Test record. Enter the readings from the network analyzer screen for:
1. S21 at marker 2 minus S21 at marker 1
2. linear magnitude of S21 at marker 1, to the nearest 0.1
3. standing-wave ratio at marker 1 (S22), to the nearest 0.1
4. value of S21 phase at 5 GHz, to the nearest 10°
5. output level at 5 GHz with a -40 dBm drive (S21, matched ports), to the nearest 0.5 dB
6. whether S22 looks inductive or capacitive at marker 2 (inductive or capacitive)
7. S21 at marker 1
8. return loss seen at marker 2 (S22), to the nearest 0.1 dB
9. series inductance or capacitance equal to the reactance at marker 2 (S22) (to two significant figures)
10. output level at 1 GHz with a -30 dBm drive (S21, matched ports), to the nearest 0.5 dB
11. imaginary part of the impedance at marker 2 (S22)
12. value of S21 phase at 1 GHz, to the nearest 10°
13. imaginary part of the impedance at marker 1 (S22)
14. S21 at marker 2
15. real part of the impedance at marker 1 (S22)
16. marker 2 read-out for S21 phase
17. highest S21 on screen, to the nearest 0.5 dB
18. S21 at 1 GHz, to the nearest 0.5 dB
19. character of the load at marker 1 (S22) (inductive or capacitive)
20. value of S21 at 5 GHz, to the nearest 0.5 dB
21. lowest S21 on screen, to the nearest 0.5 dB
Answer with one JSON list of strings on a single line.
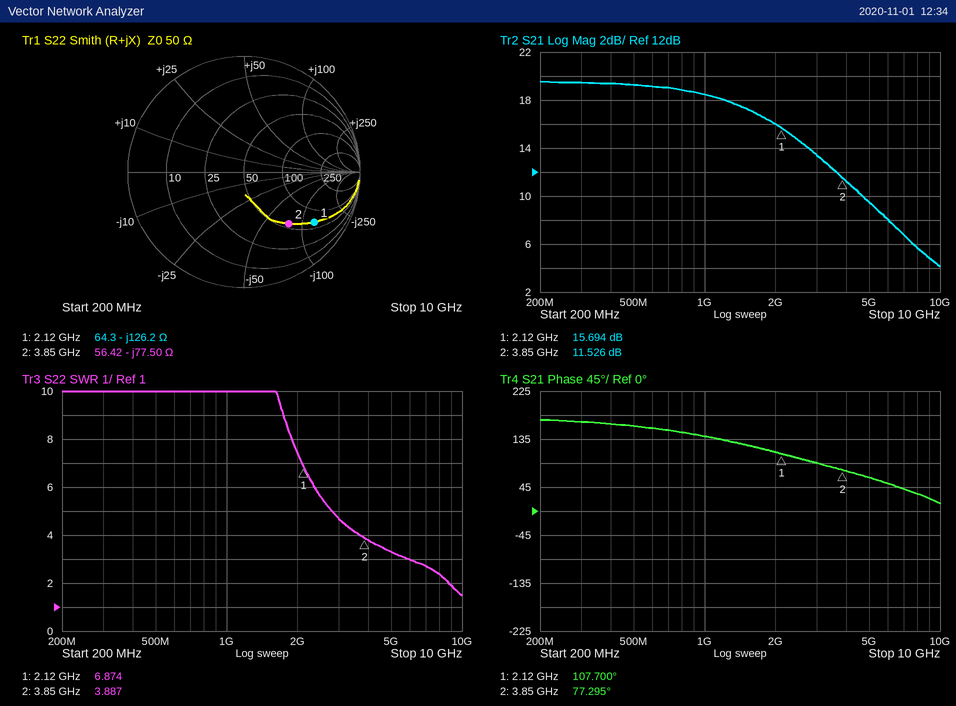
["-4.168 dB", "6.1", "6.9", "60°", "-30.5 dBm", "capacitive", "15.694 dB", "4.6 dB", "530 fF", "-11.5 dBm", "-77.50 Ω", "140°", "-126.2 Ω", "11.526 dB", "64.3 Ω", "77.295°", "19.5 dB", "18.5 dB", "capacitive", "9.5 dB", "4.0 dB"]
